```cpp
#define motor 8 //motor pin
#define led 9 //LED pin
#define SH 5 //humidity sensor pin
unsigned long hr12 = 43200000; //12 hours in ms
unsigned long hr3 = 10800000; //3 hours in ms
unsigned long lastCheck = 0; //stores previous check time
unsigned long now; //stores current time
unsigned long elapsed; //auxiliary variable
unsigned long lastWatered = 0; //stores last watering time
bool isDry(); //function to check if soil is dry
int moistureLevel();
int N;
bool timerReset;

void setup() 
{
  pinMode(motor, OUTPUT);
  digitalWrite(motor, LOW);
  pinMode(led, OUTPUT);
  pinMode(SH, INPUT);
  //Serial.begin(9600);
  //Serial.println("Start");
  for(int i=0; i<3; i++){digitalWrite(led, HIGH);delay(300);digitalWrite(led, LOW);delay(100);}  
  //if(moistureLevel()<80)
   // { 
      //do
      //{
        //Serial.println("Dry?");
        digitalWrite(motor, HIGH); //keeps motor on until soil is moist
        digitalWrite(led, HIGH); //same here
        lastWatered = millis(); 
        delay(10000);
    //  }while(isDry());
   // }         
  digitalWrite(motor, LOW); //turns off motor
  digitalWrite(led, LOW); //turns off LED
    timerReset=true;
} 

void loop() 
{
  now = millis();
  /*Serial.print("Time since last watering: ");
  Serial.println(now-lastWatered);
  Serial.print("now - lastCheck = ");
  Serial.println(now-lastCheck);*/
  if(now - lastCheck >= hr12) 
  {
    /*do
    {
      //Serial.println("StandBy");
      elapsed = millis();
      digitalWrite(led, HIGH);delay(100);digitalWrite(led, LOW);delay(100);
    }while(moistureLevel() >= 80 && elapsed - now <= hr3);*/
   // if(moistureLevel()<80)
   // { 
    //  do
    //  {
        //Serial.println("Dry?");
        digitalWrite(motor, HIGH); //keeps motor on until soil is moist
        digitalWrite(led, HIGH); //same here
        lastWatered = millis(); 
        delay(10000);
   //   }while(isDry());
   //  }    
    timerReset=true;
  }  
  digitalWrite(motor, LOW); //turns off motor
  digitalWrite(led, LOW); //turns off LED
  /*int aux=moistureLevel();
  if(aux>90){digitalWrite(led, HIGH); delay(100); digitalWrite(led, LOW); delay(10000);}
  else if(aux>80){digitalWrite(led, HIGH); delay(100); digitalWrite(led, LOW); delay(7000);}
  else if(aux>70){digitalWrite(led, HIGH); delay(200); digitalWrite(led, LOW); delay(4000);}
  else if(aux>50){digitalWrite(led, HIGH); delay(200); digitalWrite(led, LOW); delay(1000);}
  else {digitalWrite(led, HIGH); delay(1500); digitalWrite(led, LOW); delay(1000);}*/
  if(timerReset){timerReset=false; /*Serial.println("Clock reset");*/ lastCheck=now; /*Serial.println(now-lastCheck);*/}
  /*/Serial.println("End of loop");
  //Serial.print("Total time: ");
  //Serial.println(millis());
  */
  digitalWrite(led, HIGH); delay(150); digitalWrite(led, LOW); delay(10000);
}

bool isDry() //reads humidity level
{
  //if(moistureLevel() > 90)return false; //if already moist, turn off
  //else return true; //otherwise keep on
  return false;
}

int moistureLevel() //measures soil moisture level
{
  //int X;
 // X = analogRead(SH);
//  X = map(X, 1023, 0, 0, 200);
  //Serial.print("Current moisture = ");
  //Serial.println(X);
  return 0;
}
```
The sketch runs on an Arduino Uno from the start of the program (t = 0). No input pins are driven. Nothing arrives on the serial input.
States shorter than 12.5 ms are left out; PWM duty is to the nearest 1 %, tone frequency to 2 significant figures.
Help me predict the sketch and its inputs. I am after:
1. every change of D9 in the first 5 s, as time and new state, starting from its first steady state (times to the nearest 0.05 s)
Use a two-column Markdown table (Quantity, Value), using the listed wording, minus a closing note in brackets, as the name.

| Quantity | Value |
|---|---|
| every change of D9 in the first 5 s, as time and new state, starting from its first steady state | 0 s high; 0.3 s low; 0.4 s high; 0.7 s low; 0.8 s high; 1.1 s low; 1.2 s high |
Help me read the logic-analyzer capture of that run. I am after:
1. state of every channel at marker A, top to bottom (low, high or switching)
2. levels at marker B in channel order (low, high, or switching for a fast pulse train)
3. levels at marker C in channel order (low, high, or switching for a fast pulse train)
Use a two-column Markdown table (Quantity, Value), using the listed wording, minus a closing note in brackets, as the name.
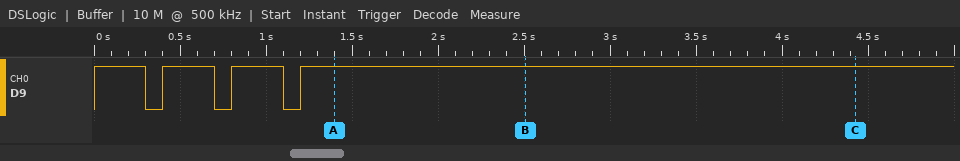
| Quantity | Value |
|---|---|
| state of every channel at marker A, top to bottom | D9 high |
| levels at marker B in channel order | D9 high |
| levels at marker C in channel order | D9 high |
